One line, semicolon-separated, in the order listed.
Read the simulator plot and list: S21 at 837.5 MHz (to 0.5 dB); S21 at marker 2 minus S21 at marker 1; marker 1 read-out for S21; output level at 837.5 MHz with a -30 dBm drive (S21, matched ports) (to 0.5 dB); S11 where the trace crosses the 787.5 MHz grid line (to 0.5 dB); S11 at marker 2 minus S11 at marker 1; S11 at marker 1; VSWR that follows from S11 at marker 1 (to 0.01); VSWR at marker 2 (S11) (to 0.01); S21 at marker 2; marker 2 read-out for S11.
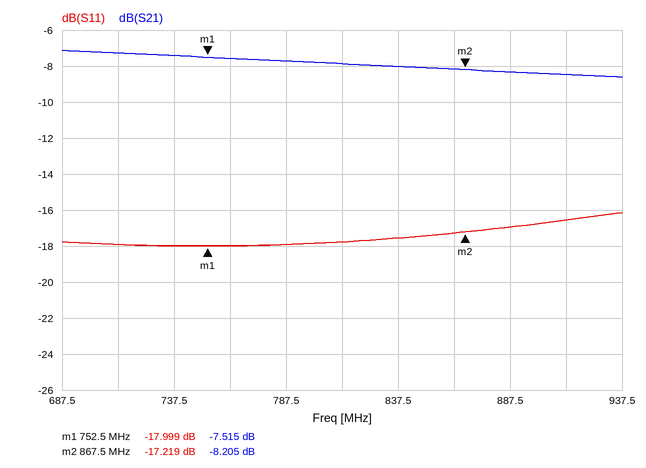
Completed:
-8.0 dB; -0.690 dB; -7.515 dB; -38.0 dBm; -18.0 dB; 0.780 dB; -17.999 dB; 1.29; 1.32; -8.205 dB; -17.219 dB
